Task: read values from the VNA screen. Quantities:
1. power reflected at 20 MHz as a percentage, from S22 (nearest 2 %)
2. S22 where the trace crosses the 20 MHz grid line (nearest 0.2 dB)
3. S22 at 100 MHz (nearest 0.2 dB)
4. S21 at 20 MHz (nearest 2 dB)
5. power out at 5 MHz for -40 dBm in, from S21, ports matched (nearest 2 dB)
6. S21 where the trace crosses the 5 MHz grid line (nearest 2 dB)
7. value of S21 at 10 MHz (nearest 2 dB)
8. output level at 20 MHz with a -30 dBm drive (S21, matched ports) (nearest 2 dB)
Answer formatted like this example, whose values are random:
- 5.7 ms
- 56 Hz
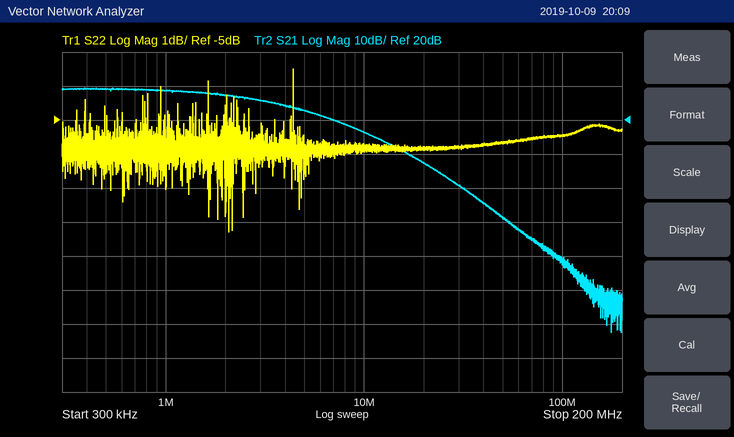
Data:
- 26 %
- -5.8 dB
- -5.4 dB
- 8 dB
- -18 dBm
- 22 dB
- 16 dB
- -22 dBm
